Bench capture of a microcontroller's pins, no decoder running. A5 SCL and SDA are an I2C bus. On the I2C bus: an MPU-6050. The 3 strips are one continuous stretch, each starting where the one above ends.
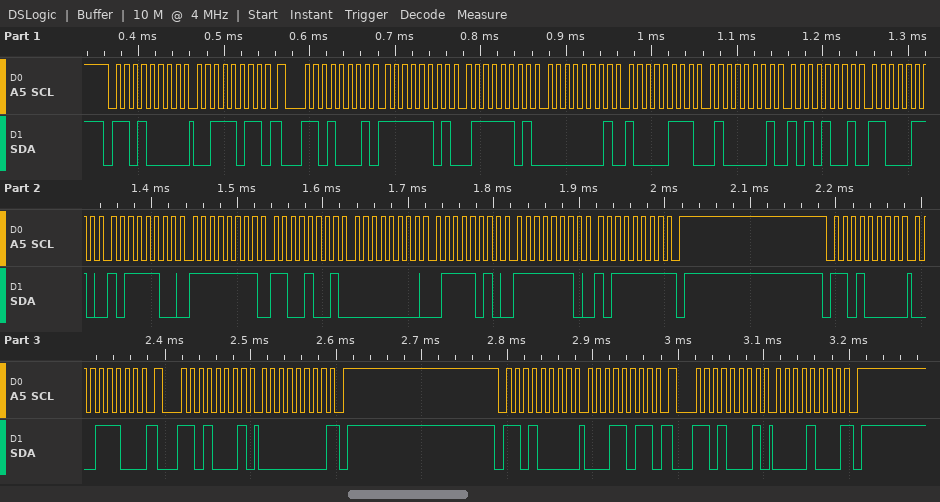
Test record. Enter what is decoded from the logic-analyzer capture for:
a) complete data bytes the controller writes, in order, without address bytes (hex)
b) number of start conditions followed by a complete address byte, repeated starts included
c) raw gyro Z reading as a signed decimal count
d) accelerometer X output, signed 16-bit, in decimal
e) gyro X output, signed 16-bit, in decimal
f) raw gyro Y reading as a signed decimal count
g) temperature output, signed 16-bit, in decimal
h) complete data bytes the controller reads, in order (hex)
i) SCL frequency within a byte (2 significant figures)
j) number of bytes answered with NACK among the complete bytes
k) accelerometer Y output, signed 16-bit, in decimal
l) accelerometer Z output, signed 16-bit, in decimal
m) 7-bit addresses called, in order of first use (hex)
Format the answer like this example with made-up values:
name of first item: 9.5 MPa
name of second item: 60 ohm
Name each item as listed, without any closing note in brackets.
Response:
complete data bytes the controller writes, in order, without address bytes: 3B 1C 1B
number of start conditions followed by a complete address byte, repeated starts included: 6
raw gyro Z reading as a signed decimal count: -321
accelerometer X output, signed 16-bit, in decimal: -643
gyro X output, signed 16-bit, in decimal: -55
raw gyro Y reading as a signed decimal count: 122
temperature output, signed 16-bit, in decimal: -14660
complete data bytes the controller reads, in order: FD 7D 01 87 41 A9 C6 BC FF C9 00 7A FE BF 00 08
SCL frequency within a byte: 100 kHz
number of bytes answered with NACK among the complete bytes: 3
accelerometer Y output, signed 16-bit, in decimal: 391
accelerometer Z output, signed 16-bit, in decimal: 16809
7-bit addresses called, in order of first use: 0x68
